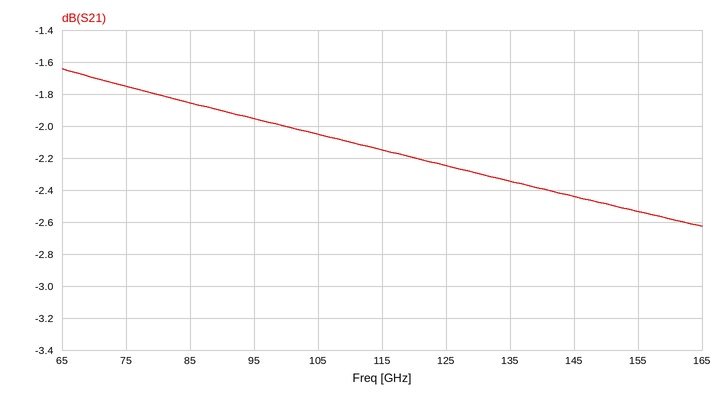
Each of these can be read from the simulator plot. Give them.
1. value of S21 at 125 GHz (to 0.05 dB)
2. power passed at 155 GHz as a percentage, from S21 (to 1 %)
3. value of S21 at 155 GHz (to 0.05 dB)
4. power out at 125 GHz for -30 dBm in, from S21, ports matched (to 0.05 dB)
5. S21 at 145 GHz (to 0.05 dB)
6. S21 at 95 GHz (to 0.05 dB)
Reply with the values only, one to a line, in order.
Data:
-2.25 dB
56 %
-2.55 dB
-32.25 dBm
-2.45 dB
-1.95 dB
